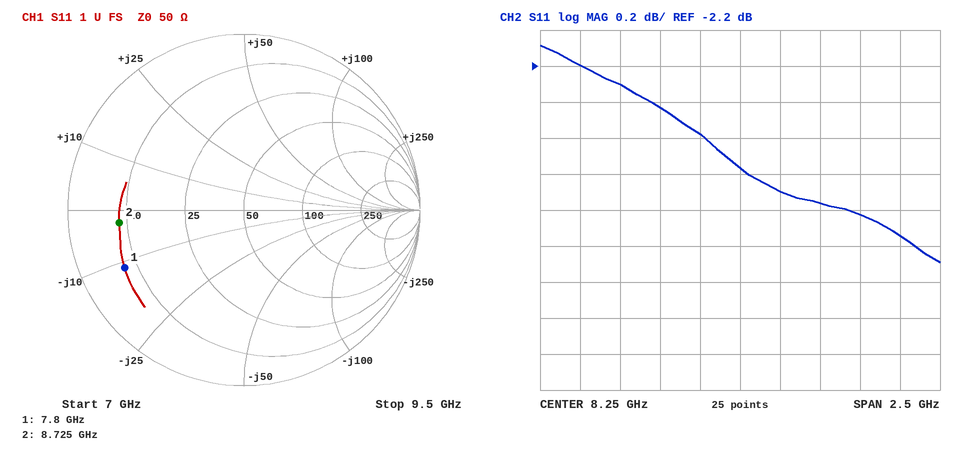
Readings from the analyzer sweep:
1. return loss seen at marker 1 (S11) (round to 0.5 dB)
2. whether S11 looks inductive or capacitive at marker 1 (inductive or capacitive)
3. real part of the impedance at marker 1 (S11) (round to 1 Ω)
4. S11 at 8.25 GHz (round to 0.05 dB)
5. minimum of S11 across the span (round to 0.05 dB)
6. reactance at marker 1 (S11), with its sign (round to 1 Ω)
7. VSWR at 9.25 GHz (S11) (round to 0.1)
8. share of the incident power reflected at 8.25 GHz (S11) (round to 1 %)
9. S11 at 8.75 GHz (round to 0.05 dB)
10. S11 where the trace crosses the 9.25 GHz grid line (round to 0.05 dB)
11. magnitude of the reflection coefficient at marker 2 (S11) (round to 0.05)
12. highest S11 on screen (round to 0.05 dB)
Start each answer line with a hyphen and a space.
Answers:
- 2.5 dB
- capacitive
- 7 Ω
- -2.75 dB
- -3.30 dB
- -11 Ω
- 5.6
- 53 %
- -2.95 dB
- -3.15 dB
- 0.70
- -2.10 dB
